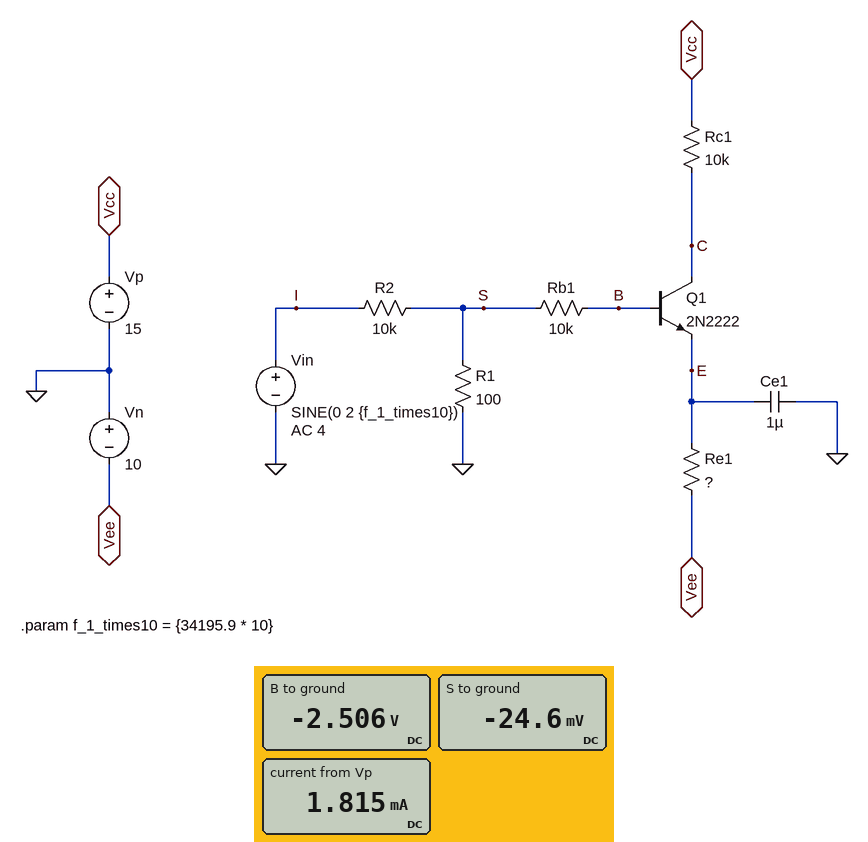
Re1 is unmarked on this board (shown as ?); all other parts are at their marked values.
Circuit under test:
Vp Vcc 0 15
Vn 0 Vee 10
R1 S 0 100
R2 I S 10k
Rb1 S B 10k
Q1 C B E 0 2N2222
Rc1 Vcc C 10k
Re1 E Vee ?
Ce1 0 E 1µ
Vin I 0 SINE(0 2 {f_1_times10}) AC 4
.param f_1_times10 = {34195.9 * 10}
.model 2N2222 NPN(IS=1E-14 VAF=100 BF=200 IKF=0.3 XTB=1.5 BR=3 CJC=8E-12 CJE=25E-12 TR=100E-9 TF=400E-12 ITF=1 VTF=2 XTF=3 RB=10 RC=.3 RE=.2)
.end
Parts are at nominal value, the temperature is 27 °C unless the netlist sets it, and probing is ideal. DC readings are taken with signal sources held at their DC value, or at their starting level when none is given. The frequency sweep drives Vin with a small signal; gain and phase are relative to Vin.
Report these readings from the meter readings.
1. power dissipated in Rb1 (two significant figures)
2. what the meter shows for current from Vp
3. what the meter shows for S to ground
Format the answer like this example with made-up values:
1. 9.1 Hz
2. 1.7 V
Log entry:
1. 620 µW
2. 1.815 mA
3. -24.6 mV
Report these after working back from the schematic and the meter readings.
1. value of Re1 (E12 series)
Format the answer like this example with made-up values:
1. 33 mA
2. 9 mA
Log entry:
1. 3.3 kΩ
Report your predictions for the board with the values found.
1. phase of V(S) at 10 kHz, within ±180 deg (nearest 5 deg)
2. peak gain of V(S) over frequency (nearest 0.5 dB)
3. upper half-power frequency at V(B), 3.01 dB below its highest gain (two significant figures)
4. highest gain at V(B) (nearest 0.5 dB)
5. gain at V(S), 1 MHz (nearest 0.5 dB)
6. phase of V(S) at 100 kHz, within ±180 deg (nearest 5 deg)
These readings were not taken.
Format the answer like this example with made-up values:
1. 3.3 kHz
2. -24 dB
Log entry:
1. 0 deg
2. -40.0 dB
3. 80 Hz
4. -54.0 dB
5. -40.0 dB
6. 0 deg
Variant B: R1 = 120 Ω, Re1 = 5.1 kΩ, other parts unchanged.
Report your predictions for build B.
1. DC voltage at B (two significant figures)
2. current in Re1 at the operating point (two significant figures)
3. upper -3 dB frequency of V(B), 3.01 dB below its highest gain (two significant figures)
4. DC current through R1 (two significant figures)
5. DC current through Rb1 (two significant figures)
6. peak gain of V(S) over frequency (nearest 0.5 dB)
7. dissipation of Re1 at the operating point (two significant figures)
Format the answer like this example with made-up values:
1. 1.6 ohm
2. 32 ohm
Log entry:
1. -680 mV
2. 1.7 mA
3. 63 Hz
4. 66 µA
5. 67 µA
6. -38.5 dB
7. 15 mW
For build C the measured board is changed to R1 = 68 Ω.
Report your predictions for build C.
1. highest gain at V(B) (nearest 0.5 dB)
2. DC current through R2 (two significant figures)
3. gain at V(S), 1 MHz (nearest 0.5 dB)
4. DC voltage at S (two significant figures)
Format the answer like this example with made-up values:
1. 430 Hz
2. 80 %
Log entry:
1. -57.5 dB
2. 1.7 µA
3. -43.5 dB
4. -17 mV
